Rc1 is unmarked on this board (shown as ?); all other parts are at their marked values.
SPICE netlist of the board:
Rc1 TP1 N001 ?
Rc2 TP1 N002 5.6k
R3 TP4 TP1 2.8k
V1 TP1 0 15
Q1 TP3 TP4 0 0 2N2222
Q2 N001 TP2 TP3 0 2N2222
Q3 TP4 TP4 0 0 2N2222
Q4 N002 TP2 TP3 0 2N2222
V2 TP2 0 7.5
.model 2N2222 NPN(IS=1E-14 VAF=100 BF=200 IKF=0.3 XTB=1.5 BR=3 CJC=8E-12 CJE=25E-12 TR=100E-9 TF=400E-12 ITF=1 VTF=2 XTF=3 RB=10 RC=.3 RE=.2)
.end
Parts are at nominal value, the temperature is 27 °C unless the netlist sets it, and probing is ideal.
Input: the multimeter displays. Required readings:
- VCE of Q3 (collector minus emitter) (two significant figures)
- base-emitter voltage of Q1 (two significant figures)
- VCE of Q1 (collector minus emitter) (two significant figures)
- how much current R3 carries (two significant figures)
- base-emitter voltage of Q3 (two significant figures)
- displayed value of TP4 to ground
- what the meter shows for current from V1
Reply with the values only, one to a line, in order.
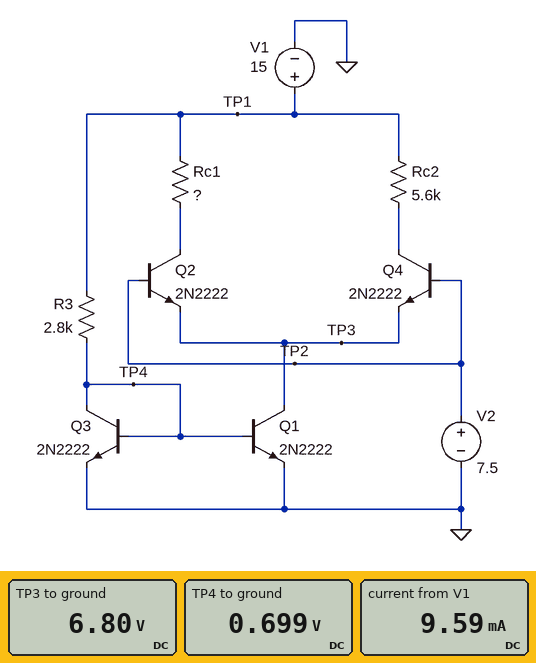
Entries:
700 mV
700 mV
6.8 V
5.1 mA
700 mV
0.699 V
9.59 mA
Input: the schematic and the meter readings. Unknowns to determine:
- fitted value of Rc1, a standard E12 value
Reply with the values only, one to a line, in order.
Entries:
2.7 kΩ
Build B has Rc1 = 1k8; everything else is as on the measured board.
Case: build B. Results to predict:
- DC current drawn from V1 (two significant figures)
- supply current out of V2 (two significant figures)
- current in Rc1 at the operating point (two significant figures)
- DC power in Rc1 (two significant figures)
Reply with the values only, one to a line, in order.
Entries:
10 mA
420 µA
3.5 mA
22 mW
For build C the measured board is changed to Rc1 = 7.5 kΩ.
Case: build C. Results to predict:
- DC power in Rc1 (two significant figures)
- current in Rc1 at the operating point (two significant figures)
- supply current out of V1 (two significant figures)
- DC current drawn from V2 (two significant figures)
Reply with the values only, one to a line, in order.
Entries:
9.0 mW
1.1 mA
7.7 mA
2.8 mA
